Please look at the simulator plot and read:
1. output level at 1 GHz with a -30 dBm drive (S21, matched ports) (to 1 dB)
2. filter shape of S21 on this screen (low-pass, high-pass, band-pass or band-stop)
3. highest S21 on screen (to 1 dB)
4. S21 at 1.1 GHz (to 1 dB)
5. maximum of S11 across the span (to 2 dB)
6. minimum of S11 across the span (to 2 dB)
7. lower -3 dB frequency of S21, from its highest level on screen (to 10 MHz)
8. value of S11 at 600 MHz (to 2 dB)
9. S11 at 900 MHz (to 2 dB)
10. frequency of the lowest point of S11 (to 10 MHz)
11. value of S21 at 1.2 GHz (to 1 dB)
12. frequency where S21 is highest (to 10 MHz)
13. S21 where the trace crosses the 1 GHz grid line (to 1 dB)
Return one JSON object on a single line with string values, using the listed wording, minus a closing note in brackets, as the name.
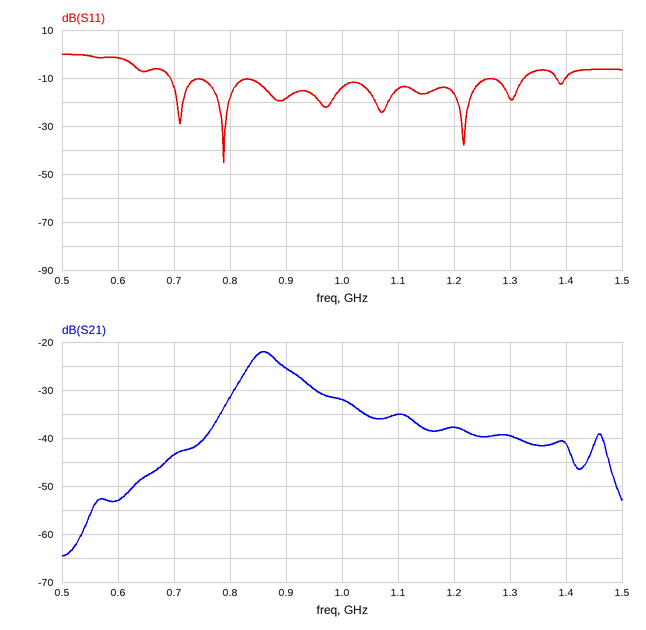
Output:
{"output level at 1 GHz with a -30 dBm drive (S21, matched ports)": "-62 dBm", "filter shape of S21 on this screen": "band-pass", "highest S21 on screen": "-22 dB", "S21 at 1.1 GHz": "-35 dB", "maximum of S11 across the span": "0 dB", "minimum of S11 across the span": "-46 dB", "lower -3 dB frequency of S21, from its highest level on screen": "830 MHz", "value of S11 at 600 MHz": "-2 dB", "S11 at 900 MHz": "-18 dB", "frequency of the lowest point of S11": "790 MHz", "value of S21 at 1.2 GHz": "-38 dB", "frequency where S21 is highest": "860 MHz", "S21 where the trace crosses the 1 GHz grid line": "-32 dB"}
